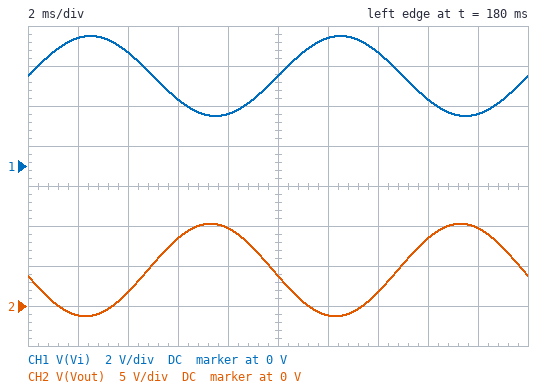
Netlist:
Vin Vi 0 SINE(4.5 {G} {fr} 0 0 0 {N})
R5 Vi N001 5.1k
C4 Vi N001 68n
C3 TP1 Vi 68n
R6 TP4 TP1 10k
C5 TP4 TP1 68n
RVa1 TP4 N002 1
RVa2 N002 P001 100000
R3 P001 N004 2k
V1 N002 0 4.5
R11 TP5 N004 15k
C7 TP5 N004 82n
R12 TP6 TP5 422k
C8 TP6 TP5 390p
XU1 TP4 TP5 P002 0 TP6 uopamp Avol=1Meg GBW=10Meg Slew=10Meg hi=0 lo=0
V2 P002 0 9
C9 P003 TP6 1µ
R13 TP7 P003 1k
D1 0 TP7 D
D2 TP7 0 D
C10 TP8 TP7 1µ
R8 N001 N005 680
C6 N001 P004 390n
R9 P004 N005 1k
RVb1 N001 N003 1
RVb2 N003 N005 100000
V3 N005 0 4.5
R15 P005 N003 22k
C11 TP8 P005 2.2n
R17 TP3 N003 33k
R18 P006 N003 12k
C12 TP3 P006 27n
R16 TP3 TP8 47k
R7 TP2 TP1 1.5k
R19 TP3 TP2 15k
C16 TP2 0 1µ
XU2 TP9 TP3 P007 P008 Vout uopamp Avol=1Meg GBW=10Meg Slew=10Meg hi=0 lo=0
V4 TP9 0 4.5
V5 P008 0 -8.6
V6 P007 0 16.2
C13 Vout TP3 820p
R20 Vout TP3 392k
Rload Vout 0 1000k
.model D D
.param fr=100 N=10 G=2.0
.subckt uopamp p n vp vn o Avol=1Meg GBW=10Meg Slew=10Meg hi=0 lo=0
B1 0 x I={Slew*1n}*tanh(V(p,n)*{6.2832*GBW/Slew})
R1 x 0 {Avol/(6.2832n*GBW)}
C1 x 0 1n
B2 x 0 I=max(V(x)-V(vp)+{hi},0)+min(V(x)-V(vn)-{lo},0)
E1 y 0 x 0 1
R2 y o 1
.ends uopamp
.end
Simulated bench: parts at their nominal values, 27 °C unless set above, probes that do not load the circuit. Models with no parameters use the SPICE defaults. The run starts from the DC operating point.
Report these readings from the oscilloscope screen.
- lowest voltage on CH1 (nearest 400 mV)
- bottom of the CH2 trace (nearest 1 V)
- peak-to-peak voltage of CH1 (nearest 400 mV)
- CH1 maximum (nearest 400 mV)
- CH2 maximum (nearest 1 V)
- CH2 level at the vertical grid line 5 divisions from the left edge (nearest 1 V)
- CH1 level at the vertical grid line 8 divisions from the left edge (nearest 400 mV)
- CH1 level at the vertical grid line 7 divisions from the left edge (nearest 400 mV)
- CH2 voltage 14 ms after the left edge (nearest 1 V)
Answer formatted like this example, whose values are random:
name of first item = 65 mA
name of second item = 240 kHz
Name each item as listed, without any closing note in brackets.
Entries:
lowest voltage on CH1 = 2.4 V
bottom of the CH2 trace = -1 V
peak-to-peak voltage of CH1 = 4.0 V
CH1 maximum = 6.4 V
CH2 maximum = 10 V
CH2 level at the vertical grid line 5 divisions from the left edge = 4 V
CH1 level at the vertical grid line 8 divisions from the left edge = 3.2 V
CH1 level at the vertical grid line 7 divisions from the left edge = 5.6 V
CH2 voltage 14 ms after the left edge = 2 V
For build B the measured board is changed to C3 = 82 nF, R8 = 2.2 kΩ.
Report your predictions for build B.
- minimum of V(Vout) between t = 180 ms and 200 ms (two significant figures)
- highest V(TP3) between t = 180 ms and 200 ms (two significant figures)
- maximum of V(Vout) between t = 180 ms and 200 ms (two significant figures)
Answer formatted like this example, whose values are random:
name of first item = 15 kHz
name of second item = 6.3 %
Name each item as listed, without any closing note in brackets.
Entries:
minimum of V(Vout) between t = 180 ms and 200 ms = -5.8 V
highest V(TP3) between t = 180 ms and 200 ms = 4.5 V
maximum of V(Vout) between t = 180 ms and 200 ms = 15 V
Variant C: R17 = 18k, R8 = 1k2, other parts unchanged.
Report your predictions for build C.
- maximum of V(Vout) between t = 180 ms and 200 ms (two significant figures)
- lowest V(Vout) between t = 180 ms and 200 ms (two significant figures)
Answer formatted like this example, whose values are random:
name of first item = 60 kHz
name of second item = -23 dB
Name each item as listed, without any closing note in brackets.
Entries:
maximum of V(Vout) between t = 180 ms and 200 ms = 15 V
lowest V(Vout) between t = 180 ms and 200 ms = -6.1 V
